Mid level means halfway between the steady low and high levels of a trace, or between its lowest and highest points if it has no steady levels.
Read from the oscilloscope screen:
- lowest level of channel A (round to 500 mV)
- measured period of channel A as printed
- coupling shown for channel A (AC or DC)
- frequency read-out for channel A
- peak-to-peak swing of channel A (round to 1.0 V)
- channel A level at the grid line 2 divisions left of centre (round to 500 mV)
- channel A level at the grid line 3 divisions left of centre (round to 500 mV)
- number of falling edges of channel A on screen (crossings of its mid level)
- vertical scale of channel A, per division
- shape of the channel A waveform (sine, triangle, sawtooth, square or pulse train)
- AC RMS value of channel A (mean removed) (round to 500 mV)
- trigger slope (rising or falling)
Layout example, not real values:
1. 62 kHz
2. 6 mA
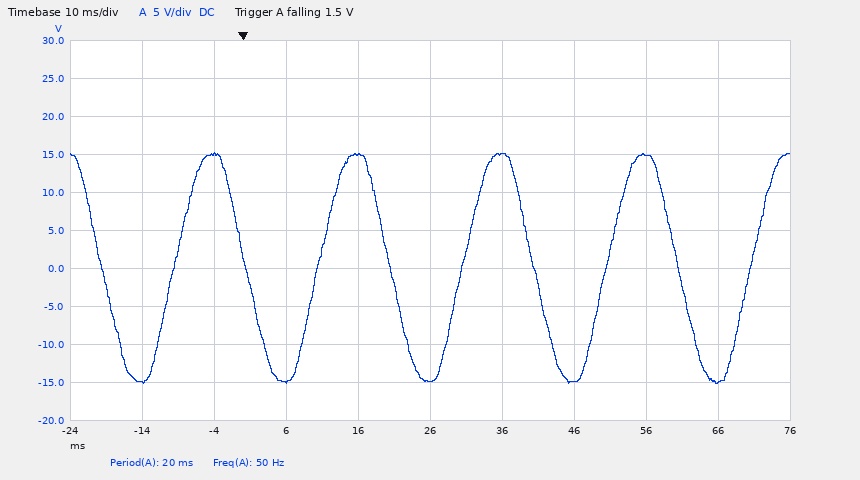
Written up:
1. -15.0 V
2. 20 ms
3. DC
4. 50 Hz
5. 30.0 V
6. -15.0 V
7. 15.0 V
8. 5
9. 5 V
10. sine
11. 10.5 V
12. falling
